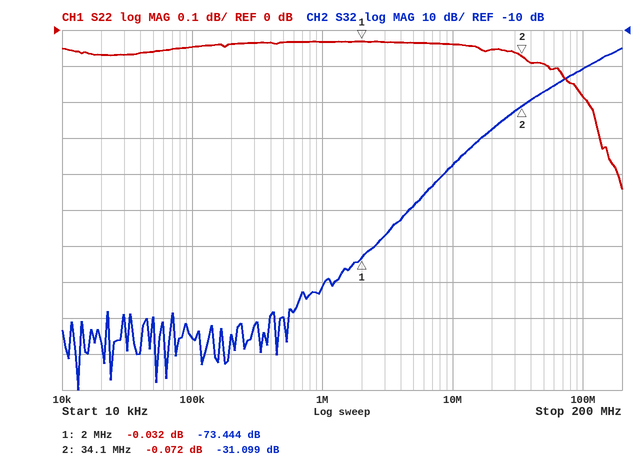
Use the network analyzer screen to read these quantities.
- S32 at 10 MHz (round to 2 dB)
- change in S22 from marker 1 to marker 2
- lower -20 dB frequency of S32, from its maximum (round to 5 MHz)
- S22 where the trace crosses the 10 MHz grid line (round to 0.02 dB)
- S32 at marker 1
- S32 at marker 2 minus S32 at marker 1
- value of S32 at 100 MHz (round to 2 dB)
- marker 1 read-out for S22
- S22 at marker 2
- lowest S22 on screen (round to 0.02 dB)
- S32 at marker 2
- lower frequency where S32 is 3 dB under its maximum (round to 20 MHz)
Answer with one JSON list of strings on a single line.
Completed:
["-48 dB", "-0.040 dB", "25 MHz", "-0.04 dB", "-73.444 dB", "42.345 dB", "-20 dB", "-0.032 dB", "-0.072 dB", "-0.44 dB", "-31.099 dB", "140 MHz"]
